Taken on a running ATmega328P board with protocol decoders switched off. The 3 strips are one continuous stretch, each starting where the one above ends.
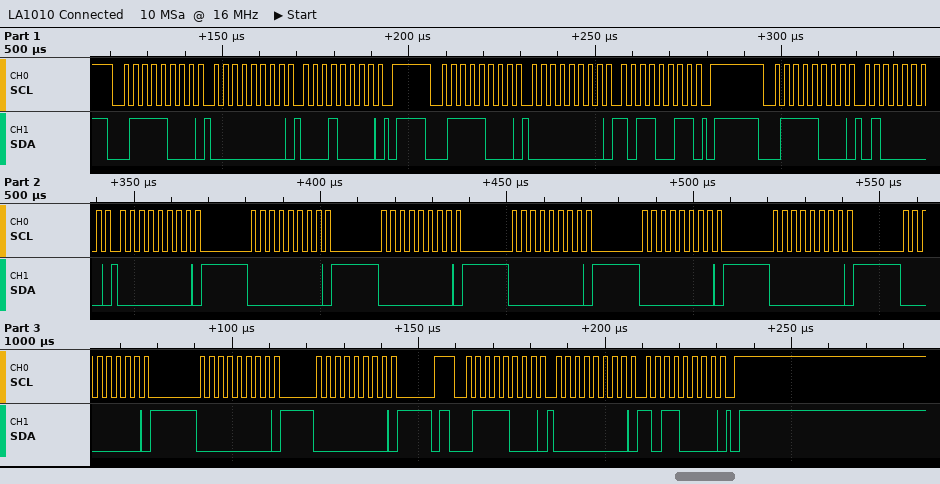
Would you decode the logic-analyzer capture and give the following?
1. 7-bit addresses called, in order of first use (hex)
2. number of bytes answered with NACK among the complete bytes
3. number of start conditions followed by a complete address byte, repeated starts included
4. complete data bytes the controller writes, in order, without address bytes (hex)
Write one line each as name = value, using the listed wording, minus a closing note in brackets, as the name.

7-bit addresses called, in order of first use = 0x3C
number of bytes answered with NACK among the complete bytes = 0
number of start conditions followed by a complete address byte, repeated starts included = 4
complete data bytes the controller writes, in order, without address bytes = 00 10 00 B3 40 00 00 00 00 00 00 00 00 00 00 B0
